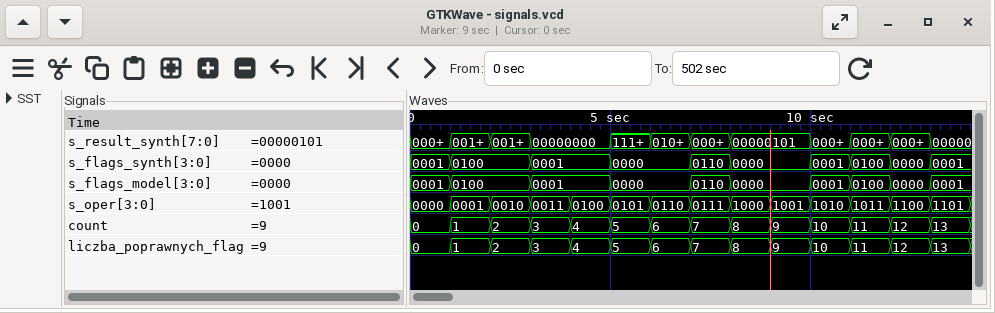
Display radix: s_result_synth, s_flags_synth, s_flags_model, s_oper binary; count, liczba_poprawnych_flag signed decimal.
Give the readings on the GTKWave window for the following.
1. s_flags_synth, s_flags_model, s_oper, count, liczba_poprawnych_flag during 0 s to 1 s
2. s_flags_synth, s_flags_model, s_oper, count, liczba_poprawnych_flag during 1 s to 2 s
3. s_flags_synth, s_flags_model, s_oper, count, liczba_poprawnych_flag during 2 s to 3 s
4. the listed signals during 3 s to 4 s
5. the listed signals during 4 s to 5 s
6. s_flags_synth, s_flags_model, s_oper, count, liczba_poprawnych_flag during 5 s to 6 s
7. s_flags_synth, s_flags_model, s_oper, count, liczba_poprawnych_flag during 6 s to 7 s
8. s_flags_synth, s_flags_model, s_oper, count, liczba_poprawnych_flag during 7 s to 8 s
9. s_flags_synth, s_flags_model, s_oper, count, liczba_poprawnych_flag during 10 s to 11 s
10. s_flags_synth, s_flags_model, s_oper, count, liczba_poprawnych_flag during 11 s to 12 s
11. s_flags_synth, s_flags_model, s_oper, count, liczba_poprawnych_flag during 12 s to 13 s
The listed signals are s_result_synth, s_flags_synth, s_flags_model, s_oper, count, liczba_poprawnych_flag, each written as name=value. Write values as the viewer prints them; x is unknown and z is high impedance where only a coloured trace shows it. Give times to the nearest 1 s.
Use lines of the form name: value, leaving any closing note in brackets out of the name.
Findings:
s_flags_synth, s_flags_model, s_oper, count, liczba_poprawnych_flag during 0 s to 1 s: s_flags_synth=0001, s_flags_model=0001, s_oper=0000, count=0, liczba_poprawnych_flag=0
s_flags_synth, s_flags_model, s_oper, count, liczba_poprawnych_flag during 1 s to 2 s: s_flags_synth=0100, s_flags_model=0100, s_oper=0001, count=1, liczba_poprawnych_flag=1
s_flags_synth, s_flags_model, s_oper, count, liczba_poprawnych_flag during 2 s to 3 s: s_flags_synth=0100, s_flags_model=0100, s_oper=0010, count=2, liczba_poprawnych_flag=2
the listed signals during 3 s to 4 s: s_result_synth=00000000, s_flags_synth=0001, s_flags_model=0001, s_oper=0011, count=3, liczba_poprawnych_flag=3
the listed signals during 4 s to 5 s: s_result_synth=00000000, s_flags_synth=0001, s_flags_model=0001, s_oper=0100, count=4, liczba_poprawnych_flag=4
s_flags_synth, s_flags_model, s_oper, count, liczba_poprawnych_flag during 5 s to 6 s: s_flags_synth=0000, s_flags_model=0000, s_oper=0101, count=5, liczba_poprawnych_flag=5
s_flags_synth, s_flags_model, s_oper, count, liczba_poprawnych_flag during 6 s to 7 s: s_flags_synth=0000, s_flags_model=0000, s_oper=0110, count=6, liczba_poprawnych_flag=6
s_flags_synth, s_flags_model, s_oper, count, liczba_poprawnych_flag during 7 s to 8 s: s_flags_synth=0110, s_flags_model=0110, s_oper=0111, count=7, liczba_poprawnych_flag=7
s_flags_synth, s_flags_model, s_oper, count, liczba_poprawnych_flag during 10 s to 11 s: s_flags_synth=0001, s_flags_model=0001, s_oper=1010, count=10, liczba_poprawnych_flag=10
s_flags_synth, s_flags_model, s_oper, count, liczba_poprawnych_flag during 11 s to 12 s: s_flags_synth=0100, s_flags_model=0100, s_oper=1011, count=11, liczba_poprawnych_flag=11
s_flags_synth, s_flags_model, s_oper, count, liczba_poprawnych_flag during 12 s to 13 s: s_flags_synth=0000, s_flags_model=0000, s_oper=1100, count=12, liczba_poprawnych_flag=12
